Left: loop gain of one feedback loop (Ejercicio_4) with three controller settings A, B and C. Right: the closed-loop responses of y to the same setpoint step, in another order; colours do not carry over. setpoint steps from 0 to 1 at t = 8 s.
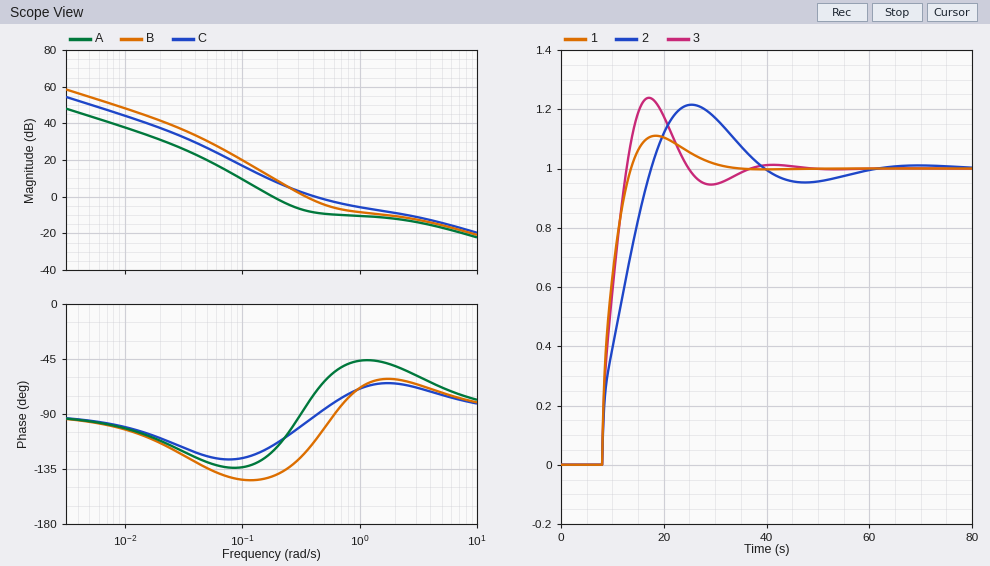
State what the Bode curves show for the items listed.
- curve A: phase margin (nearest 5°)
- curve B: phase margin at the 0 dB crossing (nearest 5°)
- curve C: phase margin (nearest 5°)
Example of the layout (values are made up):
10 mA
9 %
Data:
60°
60°
90°
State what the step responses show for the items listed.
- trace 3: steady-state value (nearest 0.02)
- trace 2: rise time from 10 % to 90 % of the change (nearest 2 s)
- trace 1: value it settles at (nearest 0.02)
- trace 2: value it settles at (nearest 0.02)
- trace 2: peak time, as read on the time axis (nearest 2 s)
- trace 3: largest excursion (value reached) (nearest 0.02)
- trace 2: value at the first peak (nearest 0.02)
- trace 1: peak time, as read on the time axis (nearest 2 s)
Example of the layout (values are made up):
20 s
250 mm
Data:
1.00
8 s
1.00
1.00
26 s
1.24
1.22
18 s
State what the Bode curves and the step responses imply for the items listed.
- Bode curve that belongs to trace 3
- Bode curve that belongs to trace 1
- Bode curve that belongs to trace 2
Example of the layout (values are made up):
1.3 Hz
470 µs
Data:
B
C
A
